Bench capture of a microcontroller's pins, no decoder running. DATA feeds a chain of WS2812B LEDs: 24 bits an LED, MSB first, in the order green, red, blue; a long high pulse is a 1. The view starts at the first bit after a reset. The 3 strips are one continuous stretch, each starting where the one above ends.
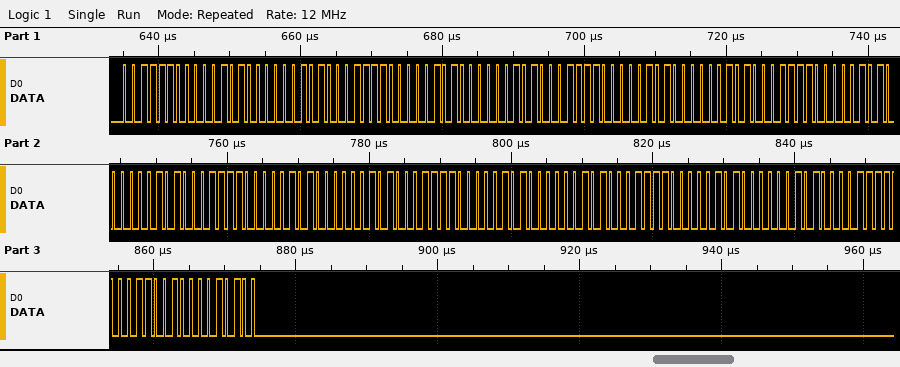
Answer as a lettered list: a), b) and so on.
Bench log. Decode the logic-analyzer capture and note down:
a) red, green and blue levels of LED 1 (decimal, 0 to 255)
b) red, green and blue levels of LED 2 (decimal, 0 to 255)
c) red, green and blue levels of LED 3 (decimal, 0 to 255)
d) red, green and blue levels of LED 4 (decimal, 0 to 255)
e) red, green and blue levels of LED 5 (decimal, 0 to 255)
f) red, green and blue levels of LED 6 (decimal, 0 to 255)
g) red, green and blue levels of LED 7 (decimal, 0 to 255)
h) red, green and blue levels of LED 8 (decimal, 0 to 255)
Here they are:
a) 20, 60, 10
b) 20, 60, 10
c) 20, 60, 10
d) 20, 60, 10
e) 20, 60, 10
f) 20, 60, 10
g) 20, 60, 10
h) 50, 30, 20
